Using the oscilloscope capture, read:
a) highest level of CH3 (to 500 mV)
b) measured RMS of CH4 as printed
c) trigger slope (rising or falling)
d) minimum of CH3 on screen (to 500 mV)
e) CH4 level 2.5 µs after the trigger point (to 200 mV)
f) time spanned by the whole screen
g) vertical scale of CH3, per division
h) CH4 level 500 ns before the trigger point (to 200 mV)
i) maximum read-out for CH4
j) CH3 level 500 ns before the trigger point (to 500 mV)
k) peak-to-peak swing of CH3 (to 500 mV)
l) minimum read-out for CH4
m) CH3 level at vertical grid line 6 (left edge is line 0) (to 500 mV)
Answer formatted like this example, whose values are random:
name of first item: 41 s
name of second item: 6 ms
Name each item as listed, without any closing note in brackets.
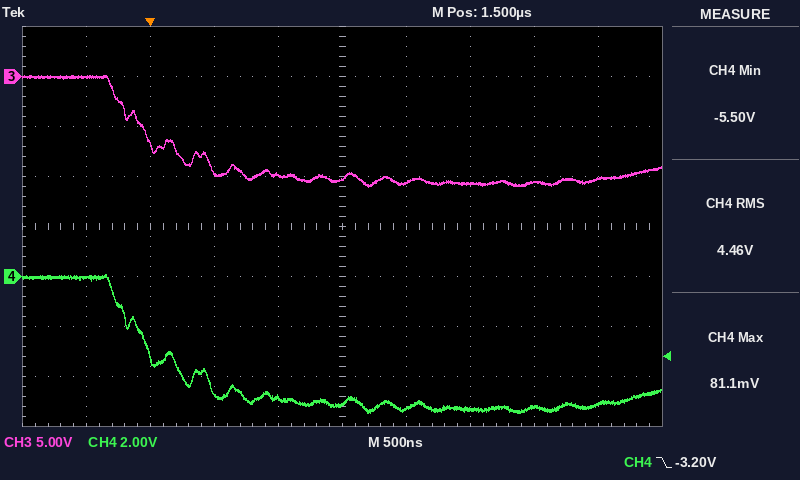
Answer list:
highest level of CH3: 0.0 V
measured RMS of CH4 as printed: 4.46 V
trigger slope: falling
minimum of CH3 on screen: -11.0 V
CH4 level 2.5 µs after the trigger point: -5.4 V
time spanned by the whole screen: 5 µs
vertical scale of CH3, per division: 5 V
CH4 level 500 ns before the trigger point: 0.0 V
maximum read-out for CH4: 81.1 mV
CH3 level 500 ns before the trigger point: 0.0 V
peak-to-peak swing of CH3: 11.0 V
minimum read-out for CH4: -5.50 V
CH3 level at vertical grid line 6 (left edge is line 0): -10.5 V
